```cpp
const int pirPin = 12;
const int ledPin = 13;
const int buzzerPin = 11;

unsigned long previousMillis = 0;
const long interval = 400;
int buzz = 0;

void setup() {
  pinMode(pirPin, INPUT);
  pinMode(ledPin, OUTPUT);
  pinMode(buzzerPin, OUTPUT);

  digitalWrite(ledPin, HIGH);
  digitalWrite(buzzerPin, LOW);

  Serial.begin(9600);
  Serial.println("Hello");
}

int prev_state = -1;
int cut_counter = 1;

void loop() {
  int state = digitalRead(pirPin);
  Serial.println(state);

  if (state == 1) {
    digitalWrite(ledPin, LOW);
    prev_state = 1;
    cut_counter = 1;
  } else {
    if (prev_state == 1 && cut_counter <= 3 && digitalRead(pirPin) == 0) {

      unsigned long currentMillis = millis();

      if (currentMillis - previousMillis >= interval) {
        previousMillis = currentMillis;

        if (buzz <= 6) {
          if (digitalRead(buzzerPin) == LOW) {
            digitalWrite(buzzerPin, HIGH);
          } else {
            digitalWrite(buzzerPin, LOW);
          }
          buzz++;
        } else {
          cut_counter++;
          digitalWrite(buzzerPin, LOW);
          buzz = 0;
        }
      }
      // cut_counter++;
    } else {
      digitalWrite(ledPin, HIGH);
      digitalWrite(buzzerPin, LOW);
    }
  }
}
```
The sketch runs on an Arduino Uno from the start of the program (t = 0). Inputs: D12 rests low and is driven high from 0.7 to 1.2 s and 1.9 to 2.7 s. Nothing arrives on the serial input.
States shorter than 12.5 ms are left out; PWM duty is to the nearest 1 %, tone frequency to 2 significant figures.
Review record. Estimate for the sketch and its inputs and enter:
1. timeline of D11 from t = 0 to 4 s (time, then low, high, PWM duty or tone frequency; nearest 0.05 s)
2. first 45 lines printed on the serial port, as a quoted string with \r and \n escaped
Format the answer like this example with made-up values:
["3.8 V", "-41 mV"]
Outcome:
["0 s low; 1.2 s high; 1.6 s low; 2.7 s high; 3.1 s low; 3.5 s high; 3.9 s low", "\"Hello\\r\\n0\\r\\n0\\r\\n0\\r\\n0\\r\\n0\\r\\n0\\r\\n0\\r\\n0\\r\\n0\\r\\n0\\r\\n0\\r\\n0\\r\\n0\\r\\n0\\r\\n0\\r\\n0\\r\\n0\\r\\n0\\r\\n0\\r\\n0\\r\\n0\\r\\n0\\r\\n0\\r\\n0\\r\\n0\\r\\n0\\r\\n0\\r\\n0\\r\\n0\\r\\n0\\r\\n0\\r\\n0\\r\\n0\\r\\n0\\r\\n0\\r\\n0\\r\\n0\\r\\n0\\r\\n0\\r\\n0\\r\\n0\\r\\n0\\r\\n0\\r\\n0\\r\\n\""]
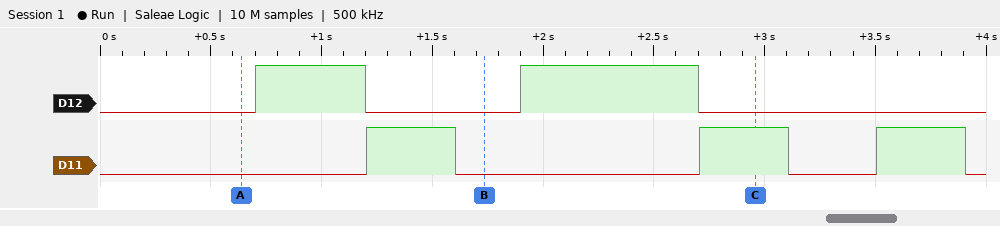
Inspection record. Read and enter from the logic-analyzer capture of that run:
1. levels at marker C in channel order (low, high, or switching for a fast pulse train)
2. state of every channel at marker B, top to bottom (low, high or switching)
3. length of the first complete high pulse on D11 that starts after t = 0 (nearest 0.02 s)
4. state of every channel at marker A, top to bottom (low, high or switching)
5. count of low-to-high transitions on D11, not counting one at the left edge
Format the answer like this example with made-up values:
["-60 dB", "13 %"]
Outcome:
["D12 low, D11 high", "D12 low, D11 low", "0.40 s", "D12 low, D11 low", "3"]
